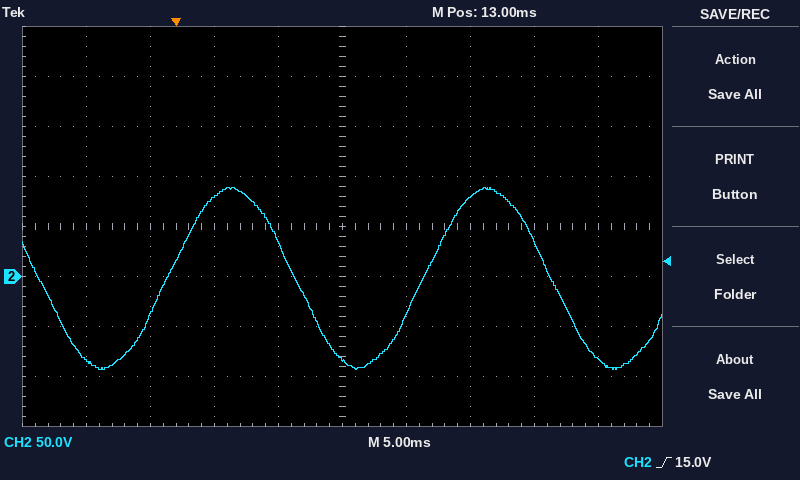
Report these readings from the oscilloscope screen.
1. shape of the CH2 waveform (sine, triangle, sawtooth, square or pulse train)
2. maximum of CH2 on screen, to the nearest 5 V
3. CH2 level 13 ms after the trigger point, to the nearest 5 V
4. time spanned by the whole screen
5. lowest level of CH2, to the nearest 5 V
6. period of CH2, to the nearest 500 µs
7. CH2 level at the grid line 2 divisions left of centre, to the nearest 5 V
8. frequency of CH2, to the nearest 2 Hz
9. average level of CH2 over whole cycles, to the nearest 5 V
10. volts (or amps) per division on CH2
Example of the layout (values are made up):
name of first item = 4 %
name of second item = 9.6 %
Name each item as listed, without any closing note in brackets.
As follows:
shape of the CH2 waveform = sine
maximum of CH2 on screen, to the nearest 5 V = 90 V
CH2 level 13 ms after the trigger point, to the nearest 5 V = -85 V
time spanned by the whole screen = 50 ms
lowest level of CH2, to the nearest 5 V = -95 V
period of CH2, to the nearest 500 µs = 20.0 ms
CH2 level at the grid line 2 divisions left of centre, to the nearest 5 V = 80 V
frequency of CH2, to the nearest 2 Hz = 50 Hz
average level of CH2 over whole cycles, to the nearest 5 V = 0 V
volts (or amps) per division on CH2 = 50 V
